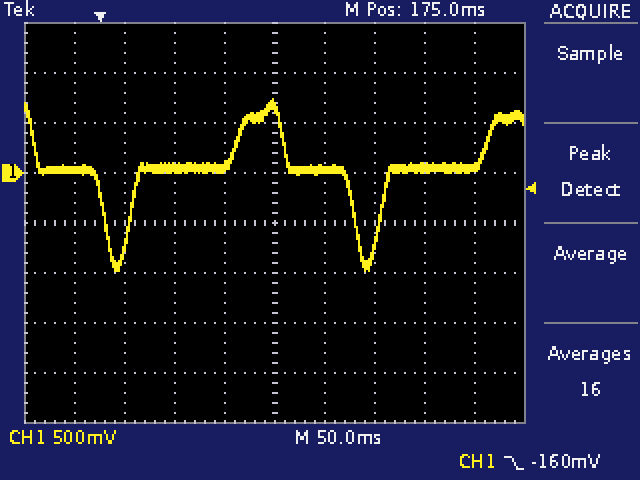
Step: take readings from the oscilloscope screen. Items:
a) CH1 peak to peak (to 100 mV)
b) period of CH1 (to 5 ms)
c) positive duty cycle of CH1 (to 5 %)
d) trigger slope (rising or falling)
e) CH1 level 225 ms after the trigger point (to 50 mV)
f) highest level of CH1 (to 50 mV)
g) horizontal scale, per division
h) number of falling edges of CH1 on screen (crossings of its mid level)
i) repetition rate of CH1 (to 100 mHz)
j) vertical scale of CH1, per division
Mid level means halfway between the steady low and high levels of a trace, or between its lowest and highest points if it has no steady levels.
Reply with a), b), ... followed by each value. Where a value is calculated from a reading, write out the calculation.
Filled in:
a) 1.70 V
b) 250 ms
c) 85 %
d) falling
e) 50 mV
f) 750 mV
g) 50 ms
h) 2
i) 1 / 250 ms ≈ 4.0 Hz
j) 500 mV
